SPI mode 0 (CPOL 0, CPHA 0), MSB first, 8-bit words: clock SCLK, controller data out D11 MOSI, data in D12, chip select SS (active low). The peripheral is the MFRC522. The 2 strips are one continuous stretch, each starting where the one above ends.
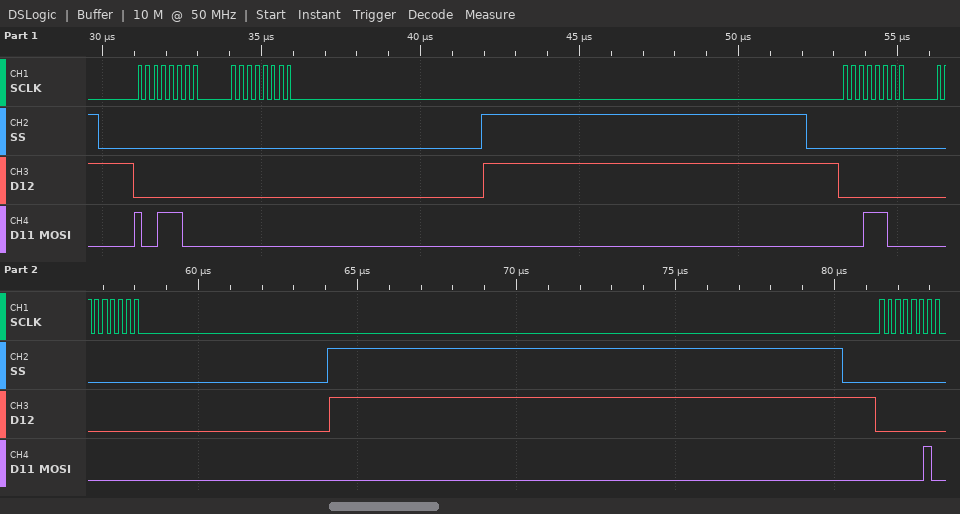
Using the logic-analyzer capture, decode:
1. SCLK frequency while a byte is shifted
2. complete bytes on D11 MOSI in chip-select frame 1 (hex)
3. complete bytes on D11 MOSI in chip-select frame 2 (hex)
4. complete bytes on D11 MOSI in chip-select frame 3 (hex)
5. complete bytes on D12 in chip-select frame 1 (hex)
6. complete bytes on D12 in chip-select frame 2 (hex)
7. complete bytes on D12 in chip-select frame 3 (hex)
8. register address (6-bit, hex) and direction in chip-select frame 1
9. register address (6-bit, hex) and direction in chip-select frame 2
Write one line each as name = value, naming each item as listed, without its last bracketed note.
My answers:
SCLK frequency while a byte is shifted = 4 MHz
complete bytes on D11 MOSI in chip-select frame 1 = 0x9C 0x00
complete bytes on D11 MOSI in chip-select frame 2 = 0x1C 0x00
complete bytes on D11 MOSI in chip-select frame 3 = 0x02
complete bytes on D12 in chip-select frame 1 = 0x00 0x00
complete bytes on D12 in chip-select frame 2 = 0x00 0x00
complete bytes on D12 in chip-select frame 3 = 0x00
register address (6-bit, hex) and direction in chip-select frame 1 = 0x0E read
register address (6-bit, hex) and direction in chip-select frame 2 = 0x0E write
